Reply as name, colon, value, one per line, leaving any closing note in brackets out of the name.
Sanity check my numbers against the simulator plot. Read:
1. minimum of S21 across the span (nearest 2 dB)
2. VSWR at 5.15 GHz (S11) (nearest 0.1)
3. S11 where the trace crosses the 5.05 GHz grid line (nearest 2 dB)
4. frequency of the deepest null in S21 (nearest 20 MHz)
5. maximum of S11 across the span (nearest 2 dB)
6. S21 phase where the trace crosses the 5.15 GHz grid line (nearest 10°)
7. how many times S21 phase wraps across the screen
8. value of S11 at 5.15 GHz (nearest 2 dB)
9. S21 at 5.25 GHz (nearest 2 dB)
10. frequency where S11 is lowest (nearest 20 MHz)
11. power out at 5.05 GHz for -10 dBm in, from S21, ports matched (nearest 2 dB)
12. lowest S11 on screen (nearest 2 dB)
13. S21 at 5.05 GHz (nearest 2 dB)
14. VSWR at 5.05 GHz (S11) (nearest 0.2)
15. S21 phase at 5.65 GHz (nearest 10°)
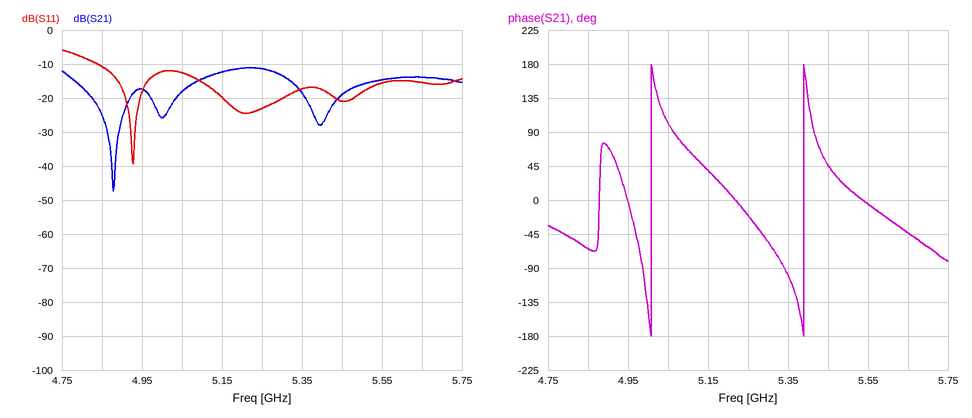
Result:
minimum of S21 across the span: -48 dB
VSWR at 5.15 GHz (S11): 1.2
S11 where the trace crosses the 5.05 GHz grid line: -12 dB
frequency of the deepest null in S21: 4.88 GHz
maximum of S11 across the span: -6 dB
S21 phase where the trace crosses the 5.15 GHz grid line: 40°
how many times S21 phase wraps across the screen: 2
value of S11 at 5.15 GHz: -20 dB
S21 at 5.25 GHz: -12 dB
frequency where S11 is lowest: 4.92 GHz
power out at 5.05 GHz for -10 dBm in, from S21, ports matched: -28 dBm
lowest S11 on screen: -40 dB
S21 at 5.05 GHz: -18 dB
VSWR at 5.05 GHz (S11): 1.6
S21 phase at 5.65 GHz: -40°
